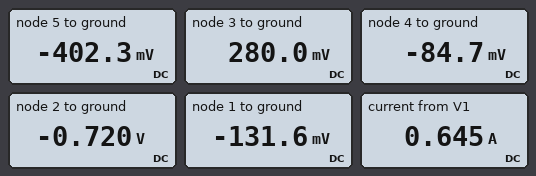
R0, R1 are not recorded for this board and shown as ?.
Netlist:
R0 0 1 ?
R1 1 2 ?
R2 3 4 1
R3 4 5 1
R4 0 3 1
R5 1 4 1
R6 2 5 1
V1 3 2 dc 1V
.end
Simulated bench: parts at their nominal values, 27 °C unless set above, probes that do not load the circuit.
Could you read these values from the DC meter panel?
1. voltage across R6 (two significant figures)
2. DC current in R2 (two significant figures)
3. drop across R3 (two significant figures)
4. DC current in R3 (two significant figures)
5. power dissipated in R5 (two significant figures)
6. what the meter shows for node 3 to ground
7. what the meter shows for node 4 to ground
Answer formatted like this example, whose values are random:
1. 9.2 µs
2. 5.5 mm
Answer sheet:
1. 320 mV
2. 360 mA
3. 320 mV
4. 320 mA
5. 2.2 mW
6. 280.0 mV
7. -84.7 mV
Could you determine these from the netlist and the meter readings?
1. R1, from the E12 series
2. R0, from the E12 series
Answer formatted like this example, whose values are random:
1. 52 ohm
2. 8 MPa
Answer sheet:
1. 1.8 Ω
2. 0.47 Ω
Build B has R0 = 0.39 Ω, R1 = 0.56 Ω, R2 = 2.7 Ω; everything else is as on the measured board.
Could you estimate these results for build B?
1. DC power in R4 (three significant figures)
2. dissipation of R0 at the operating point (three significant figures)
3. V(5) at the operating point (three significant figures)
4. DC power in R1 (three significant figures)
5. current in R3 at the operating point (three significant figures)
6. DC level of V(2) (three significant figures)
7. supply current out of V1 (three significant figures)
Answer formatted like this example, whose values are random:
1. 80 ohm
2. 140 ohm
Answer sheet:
1. 247 mW
2. 96.4 mW
3. -321 mV
4. 170 mW
5. 182 mA
6. -503 mV
7. 733 mA
